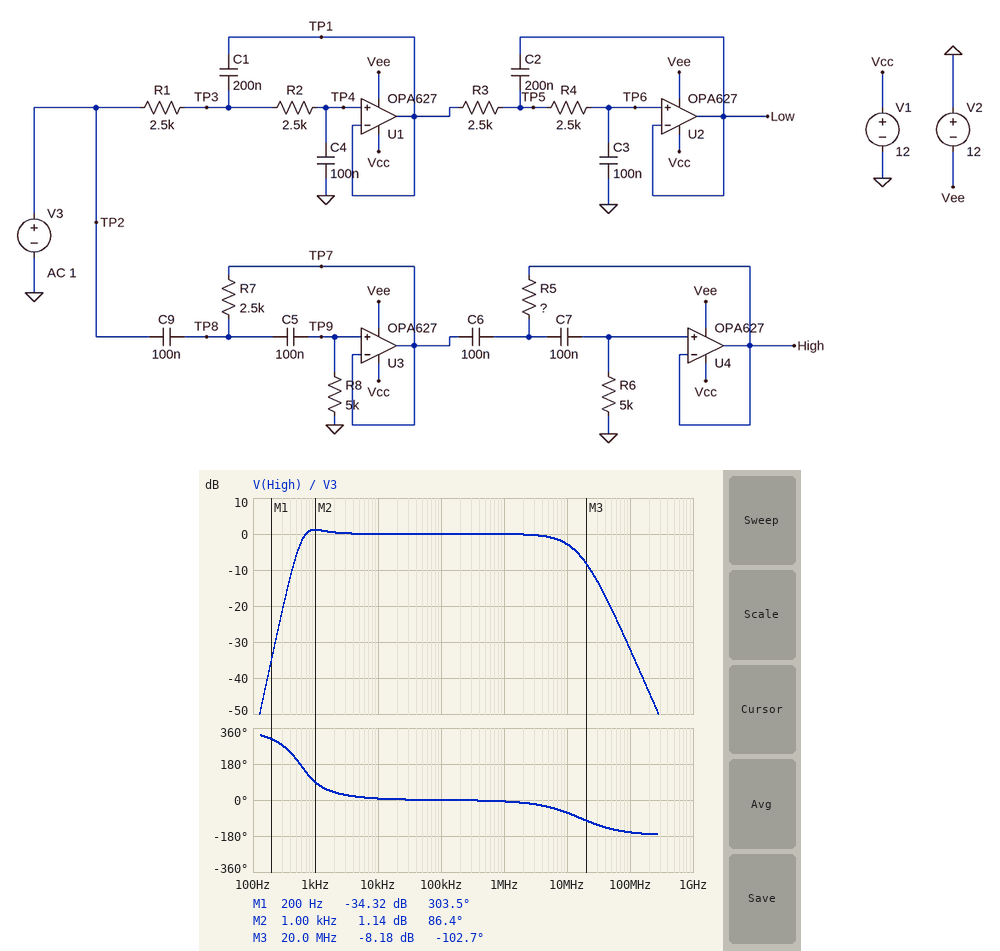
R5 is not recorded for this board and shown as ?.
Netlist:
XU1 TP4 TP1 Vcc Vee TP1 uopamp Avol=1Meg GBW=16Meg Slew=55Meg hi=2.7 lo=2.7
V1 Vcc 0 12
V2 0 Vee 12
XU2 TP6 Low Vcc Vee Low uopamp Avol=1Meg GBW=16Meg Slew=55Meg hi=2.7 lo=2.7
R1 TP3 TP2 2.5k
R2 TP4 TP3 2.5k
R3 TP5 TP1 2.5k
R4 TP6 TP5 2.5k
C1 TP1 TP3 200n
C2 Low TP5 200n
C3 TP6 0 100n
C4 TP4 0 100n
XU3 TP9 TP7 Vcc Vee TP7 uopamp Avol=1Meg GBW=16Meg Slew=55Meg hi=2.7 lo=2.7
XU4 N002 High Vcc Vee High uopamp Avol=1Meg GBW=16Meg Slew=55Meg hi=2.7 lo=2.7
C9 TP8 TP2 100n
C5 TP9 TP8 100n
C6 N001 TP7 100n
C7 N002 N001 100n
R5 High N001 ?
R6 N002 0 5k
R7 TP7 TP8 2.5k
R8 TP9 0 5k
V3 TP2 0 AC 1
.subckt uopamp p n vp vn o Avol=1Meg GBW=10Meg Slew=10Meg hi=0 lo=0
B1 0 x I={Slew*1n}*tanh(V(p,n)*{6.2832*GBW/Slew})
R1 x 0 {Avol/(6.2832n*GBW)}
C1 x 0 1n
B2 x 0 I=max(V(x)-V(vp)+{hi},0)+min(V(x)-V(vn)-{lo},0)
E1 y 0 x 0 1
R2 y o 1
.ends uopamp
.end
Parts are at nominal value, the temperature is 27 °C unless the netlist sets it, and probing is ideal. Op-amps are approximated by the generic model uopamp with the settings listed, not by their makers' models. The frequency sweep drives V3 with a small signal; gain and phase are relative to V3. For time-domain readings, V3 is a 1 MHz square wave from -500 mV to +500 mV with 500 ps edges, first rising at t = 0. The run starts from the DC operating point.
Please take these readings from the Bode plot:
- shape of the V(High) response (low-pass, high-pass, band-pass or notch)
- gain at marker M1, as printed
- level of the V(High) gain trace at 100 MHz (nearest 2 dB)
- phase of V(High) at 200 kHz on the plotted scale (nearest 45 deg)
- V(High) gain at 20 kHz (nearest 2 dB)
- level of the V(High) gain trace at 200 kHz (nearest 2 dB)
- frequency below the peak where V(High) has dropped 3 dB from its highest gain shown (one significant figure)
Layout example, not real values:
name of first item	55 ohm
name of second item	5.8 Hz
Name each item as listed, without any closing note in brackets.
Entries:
shape of the V(High) response	band-pass
gain at marker M1, as printed	-34.32 dB
level of the V(High) gain trace at 100 MHz	-32 dB
phase of V(High) at 200 kHz on the plotted scale	0 deg
V(High) gain at 20 kHz	0 dB
level of the V(High) gain trace at 200 kHz	0 dB
frequency below the peak where V(High) has dropped 3 dB from its highest gain shown	600 Hz
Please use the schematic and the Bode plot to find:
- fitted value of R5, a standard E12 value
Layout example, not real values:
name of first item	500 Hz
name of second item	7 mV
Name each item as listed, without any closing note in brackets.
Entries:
fitted value of R5, a standard E12 value	1.2 kΩ
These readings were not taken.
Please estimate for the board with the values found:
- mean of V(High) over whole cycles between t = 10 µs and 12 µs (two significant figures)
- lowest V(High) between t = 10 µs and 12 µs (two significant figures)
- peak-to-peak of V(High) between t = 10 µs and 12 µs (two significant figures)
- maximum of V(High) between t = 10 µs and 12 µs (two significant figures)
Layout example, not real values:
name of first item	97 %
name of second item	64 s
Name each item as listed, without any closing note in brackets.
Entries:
mean of V(High) over whole cycles between t = 10 µs and 12 µs	460 mV
lowest V(High) between t = 10 µs and 12 µs	-47 mV
peak-to-peak of V(High) between t = 10 µs and 12 µs	1.0 V
maximum of V(High) between t = 10 µs and 12 µs	960 mV
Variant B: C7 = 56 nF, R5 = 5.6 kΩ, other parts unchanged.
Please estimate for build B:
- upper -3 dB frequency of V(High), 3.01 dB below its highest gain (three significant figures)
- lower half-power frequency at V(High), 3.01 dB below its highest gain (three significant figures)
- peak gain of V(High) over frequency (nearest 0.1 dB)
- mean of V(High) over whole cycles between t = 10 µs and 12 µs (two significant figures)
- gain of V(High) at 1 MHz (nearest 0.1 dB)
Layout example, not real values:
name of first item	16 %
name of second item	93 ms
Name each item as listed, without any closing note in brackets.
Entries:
upper -3 dB frequency of V(High), 3.01 dB below its highest gain	10.3 MHz
lower half-power frequency at V(High), 3.01 dB below its highest gain	790 Hz
peak gain of V(High) over frequency	0 dB
mean of V(High) over whole cycles between t = 10 µs and 12 µs	450 mV
gain of V(High) at 1 MHz	0 dB
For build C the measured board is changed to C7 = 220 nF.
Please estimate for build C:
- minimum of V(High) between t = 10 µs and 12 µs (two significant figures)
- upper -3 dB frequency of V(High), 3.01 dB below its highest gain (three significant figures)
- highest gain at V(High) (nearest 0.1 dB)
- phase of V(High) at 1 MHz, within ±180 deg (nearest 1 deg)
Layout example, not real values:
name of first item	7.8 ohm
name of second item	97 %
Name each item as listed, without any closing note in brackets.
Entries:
minimum of V(High) between t = 10 µs and 12 µs	-41 mV
upper -3 dB frequency of V(High), 3.01 dB below its highest gain	9.35 MHz
highest gain at V(High)	0.5 dB
phase of V(High) at 1 MHz, within ±180 deg	-7 deg
